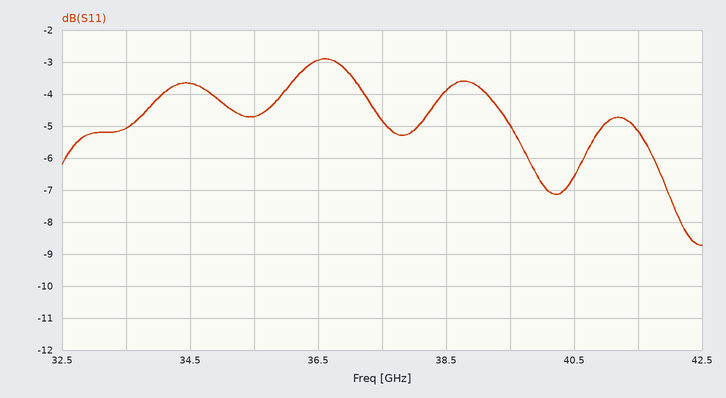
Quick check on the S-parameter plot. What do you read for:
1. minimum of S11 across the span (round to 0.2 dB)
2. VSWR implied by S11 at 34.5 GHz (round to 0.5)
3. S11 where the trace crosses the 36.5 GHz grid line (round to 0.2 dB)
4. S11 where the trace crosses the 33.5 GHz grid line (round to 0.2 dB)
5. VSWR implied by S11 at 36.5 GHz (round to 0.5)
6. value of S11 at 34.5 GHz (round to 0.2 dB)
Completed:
-8.8 dB
5.0
-3.0 dB
-5.0 dB
6.0
-3.6 dB
